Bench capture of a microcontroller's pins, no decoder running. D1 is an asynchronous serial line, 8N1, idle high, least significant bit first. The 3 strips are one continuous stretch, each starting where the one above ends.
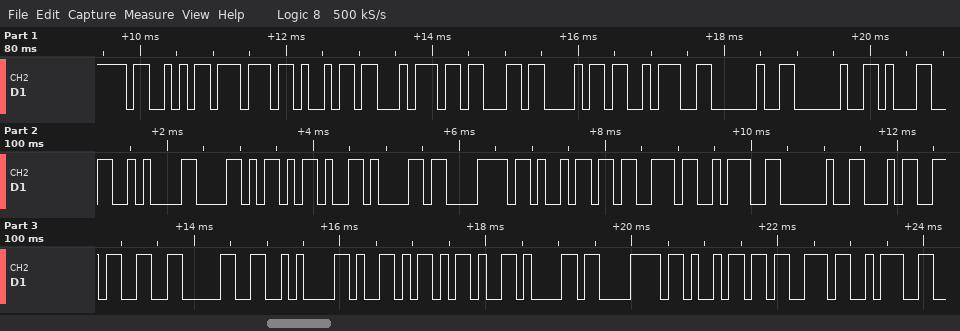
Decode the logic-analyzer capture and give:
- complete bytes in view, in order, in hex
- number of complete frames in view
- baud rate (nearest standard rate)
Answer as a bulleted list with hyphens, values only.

- 53 77 69 74 63 68 3A 20 20 31 0A 58 2D 61 78 69 73 3A 20 34 33 30 0A 59 2D 61 78 69 73 3A
- 30
- 9600 baud
